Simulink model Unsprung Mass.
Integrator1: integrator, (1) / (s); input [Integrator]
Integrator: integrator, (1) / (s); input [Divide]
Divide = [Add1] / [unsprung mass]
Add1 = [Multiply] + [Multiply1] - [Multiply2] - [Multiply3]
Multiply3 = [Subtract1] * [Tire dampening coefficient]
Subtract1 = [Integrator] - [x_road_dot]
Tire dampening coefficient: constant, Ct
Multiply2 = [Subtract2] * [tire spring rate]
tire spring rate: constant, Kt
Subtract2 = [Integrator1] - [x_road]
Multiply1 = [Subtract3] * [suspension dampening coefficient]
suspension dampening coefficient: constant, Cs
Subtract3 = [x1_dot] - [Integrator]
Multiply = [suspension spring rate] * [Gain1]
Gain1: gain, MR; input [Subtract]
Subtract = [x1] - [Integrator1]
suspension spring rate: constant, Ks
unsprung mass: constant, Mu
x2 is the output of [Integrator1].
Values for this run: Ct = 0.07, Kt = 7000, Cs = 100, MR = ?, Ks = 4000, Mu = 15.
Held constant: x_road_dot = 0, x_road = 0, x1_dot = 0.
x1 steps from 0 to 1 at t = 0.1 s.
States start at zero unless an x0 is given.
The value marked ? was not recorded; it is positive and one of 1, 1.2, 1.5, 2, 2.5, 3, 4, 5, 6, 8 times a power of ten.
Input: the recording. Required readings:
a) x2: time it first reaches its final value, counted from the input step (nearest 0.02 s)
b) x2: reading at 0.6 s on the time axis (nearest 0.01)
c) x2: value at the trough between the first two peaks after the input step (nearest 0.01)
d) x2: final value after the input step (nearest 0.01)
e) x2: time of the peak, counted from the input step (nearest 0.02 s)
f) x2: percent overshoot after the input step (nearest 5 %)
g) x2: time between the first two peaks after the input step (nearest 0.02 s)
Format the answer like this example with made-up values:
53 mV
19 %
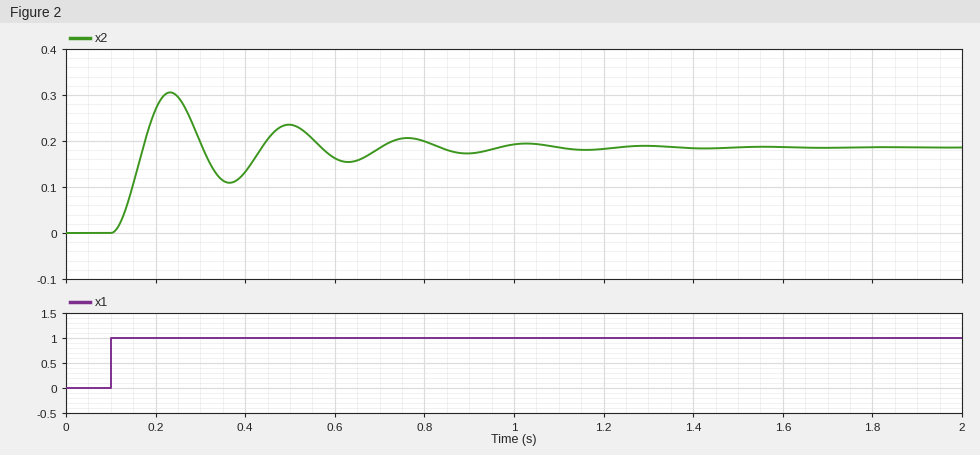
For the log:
0.08 s
0.16
0.11
0.19
0.14 s
65 %
0.26 s
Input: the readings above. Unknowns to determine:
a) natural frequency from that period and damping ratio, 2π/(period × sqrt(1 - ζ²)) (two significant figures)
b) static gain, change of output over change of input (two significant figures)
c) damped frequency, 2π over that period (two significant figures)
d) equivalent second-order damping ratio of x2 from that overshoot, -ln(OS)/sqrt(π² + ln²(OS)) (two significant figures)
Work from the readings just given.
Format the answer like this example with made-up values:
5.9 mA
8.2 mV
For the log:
24 rad/s
0.19
24 rad/s
0.14
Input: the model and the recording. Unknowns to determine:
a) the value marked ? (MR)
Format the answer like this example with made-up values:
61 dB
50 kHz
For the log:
0.4
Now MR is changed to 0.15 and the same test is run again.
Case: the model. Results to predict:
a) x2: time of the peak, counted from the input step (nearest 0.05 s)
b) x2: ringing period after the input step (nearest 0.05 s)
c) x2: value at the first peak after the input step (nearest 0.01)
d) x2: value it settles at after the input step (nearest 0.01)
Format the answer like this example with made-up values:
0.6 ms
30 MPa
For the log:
0.15 s
0.30 s
0.13
0.08
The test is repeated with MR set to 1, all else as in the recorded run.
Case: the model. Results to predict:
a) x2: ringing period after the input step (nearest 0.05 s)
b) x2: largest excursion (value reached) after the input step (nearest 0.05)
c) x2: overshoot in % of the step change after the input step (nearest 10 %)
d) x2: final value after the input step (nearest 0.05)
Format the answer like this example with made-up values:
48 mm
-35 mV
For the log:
0.25 s
0.60
70 %
0.35
